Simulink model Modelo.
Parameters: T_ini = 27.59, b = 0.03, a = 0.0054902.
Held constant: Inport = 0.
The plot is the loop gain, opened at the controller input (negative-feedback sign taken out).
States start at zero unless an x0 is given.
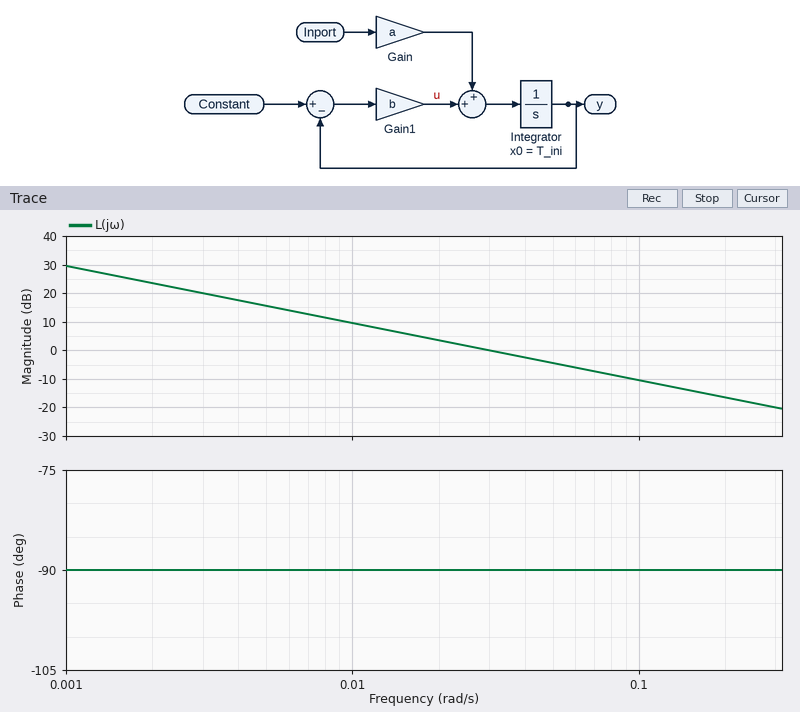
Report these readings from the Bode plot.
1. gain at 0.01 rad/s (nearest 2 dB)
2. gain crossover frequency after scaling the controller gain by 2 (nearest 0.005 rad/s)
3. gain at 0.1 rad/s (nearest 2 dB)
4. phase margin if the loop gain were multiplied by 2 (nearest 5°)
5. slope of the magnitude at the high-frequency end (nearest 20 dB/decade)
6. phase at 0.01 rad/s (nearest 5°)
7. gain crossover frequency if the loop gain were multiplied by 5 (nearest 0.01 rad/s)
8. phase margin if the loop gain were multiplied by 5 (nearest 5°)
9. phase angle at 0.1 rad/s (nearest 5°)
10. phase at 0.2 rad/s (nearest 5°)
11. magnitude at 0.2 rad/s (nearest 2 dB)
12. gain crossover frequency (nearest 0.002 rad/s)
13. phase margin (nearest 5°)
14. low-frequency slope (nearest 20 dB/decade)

10 dB
0.060 rad/s
-10 dB
90°
-20 dB/decade
-90°
0.15 rad/s
90°
-90°
-90°
-16 dB
0.030 rad/s
90°
-20 dB/decade
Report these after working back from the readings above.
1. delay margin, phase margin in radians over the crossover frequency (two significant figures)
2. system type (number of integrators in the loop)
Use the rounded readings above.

52 s
1
